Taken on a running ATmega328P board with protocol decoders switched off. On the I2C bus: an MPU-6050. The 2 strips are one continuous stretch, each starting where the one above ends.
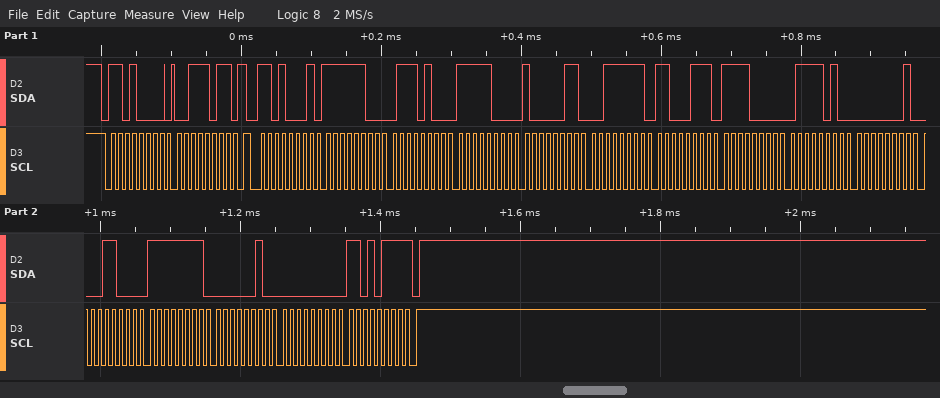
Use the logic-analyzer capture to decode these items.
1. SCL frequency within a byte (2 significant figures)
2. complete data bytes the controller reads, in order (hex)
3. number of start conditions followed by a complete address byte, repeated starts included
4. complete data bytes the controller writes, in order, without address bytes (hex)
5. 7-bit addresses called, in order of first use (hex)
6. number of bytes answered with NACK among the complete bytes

100 kHz
FC 74 F8 83 3F C7 F0 7A 01 18 FF 02 00 D7
2
3B
0x68
1
